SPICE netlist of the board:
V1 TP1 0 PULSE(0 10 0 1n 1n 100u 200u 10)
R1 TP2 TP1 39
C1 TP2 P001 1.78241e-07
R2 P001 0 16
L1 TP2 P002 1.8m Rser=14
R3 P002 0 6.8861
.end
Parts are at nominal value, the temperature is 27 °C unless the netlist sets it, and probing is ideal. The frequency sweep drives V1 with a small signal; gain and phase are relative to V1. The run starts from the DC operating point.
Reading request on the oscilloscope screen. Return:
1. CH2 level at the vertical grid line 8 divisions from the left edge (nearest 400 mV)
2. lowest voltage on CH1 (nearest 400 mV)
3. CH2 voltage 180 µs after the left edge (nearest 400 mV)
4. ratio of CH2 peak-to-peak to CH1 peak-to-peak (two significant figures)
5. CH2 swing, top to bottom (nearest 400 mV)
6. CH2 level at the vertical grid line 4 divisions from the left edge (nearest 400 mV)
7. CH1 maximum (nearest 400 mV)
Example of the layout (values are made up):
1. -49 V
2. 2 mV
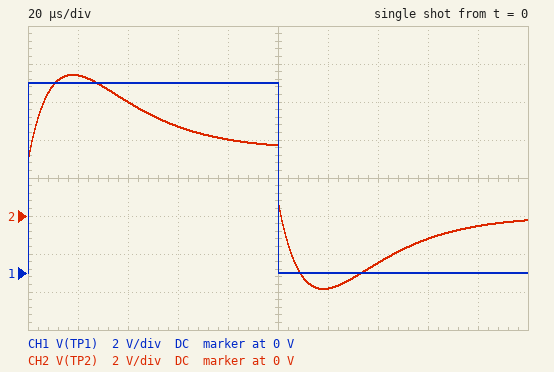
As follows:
1. -1.2 V
2. 0 V
3. -400 mV
4. 1.1
5. 11.2 V
6. 4.0 V
7. 10.0 V
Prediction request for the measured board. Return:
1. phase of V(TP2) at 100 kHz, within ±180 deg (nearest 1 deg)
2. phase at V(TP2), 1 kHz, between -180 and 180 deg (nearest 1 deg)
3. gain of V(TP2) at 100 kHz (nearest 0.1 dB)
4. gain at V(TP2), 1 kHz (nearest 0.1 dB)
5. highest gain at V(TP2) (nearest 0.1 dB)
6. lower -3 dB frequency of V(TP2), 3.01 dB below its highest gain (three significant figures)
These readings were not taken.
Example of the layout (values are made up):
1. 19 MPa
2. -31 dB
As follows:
1. -19 deg
2. 17 deg
3. -9.6 dB
4. -8.1 dB
5. -1.1 dB
6. 3.24 kHz
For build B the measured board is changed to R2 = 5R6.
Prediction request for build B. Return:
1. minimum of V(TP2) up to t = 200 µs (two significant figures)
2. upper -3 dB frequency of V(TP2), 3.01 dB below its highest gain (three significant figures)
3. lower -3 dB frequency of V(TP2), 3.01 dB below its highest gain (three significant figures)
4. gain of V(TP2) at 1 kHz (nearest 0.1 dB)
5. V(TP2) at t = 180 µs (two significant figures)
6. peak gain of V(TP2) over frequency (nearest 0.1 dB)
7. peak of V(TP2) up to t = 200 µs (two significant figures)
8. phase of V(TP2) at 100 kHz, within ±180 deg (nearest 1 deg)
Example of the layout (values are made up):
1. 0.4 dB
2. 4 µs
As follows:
1. -4.2 V
2. 26.2 kHz
3. 3.47 kHz
4. -8.1 dB
5. -500 mV
6. -0.8 dB
7. 7.8 V
8. -46 deg
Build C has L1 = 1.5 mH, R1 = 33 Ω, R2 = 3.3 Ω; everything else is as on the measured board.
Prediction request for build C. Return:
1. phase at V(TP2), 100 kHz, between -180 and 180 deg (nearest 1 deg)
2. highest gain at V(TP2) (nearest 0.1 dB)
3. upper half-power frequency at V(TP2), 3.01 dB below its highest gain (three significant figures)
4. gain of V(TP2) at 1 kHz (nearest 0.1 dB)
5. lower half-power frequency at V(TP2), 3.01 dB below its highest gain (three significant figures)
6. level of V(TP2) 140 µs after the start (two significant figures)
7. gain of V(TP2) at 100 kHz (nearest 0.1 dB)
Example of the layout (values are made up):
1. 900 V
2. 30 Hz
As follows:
1. -56 deg
2. -0.7 dB
3. 31.1 kHz
4. -7.5 dB
5. 3.67 kHz
6. -2.0 V
7. -11.8 dB
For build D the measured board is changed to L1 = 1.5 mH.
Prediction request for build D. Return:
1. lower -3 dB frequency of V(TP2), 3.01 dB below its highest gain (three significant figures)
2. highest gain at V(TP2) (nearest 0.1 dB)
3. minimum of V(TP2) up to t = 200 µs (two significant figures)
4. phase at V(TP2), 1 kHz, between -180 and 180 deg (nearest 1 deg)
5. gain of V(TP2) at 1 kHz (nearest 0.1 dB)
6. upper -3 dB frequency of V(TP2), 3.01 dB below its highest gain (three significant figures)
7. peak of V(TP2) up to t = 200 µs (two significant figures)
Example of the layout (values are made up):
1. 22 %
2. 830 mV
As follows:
1. 3.69 kHz
2. -1.3 dB
3. -3.7 V
4. 14 deg
5. -8.4 dB
6. 26.1 kHz
7. 7.2 V
